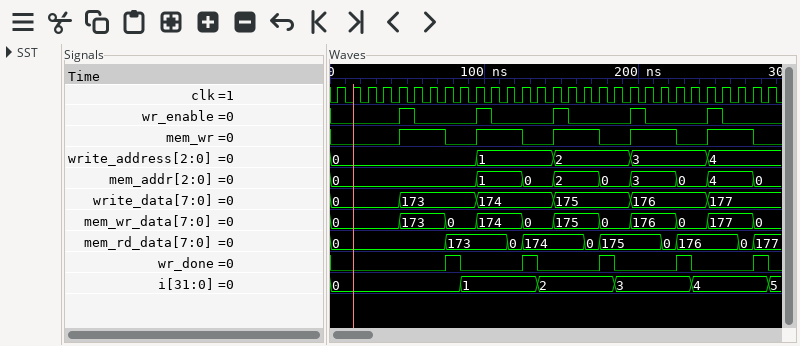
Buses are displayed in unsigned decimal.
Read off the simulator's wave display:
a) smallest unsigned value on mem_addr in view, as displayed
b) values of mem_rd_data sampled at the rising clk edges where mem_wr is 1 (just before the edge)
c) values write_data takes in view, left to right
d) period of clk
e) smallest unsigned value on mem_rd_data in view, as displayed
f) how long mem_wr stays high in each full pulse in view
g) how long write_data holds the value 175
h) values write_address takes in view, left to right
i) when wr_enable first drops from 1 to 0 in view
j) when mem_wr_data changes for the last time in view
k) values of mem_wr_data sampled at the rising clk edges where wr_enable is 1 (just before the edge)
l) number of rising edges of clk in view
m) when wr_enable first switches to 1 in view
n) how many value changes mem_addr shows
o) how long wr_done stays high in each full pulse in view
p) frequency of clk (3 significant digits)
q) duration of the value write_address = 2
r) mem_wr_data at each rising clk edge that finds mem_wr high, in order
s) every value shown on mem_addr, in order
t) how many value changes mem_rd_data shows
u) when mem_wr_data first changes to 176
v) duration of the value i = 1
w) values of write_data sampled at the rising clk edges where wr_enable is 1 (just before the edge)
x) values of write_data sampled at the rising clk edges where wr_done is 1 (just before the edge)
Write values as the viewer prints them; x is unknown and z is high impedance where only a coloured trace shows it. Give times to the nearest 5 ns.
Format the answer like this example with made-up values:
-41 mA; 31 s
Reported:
0; 0, 0, 0, 173, 173, 0, 174, 174, 0, 175, 175, 0, 176, 176, 0; 0, 173, 174, 175, 176, 177; 10 ns; 0; 30 ns, 30 ns, 30 ns, 30 ns, 30 ns; 50 ns; 0, 1, 2, 3, 4; 55 ns; 275 ns; 173, 174, 175, 176, 177; 29; 45 ns; 8; 10 ns, 10 ns, 10 ns, 10 ns, 10 ns; 100 MHz; 50 ns; 173, 173, 173, 174, 174, 174, 175, 175, 175, 176, 176, 176, 177, 177, 177; 0, 1, 0, 2, 0, 3, 0, 4, 0; 9; 195 ns; 50 ns; 173, 174, 175, 176, 177; 173, 174, 175, 176, 177
